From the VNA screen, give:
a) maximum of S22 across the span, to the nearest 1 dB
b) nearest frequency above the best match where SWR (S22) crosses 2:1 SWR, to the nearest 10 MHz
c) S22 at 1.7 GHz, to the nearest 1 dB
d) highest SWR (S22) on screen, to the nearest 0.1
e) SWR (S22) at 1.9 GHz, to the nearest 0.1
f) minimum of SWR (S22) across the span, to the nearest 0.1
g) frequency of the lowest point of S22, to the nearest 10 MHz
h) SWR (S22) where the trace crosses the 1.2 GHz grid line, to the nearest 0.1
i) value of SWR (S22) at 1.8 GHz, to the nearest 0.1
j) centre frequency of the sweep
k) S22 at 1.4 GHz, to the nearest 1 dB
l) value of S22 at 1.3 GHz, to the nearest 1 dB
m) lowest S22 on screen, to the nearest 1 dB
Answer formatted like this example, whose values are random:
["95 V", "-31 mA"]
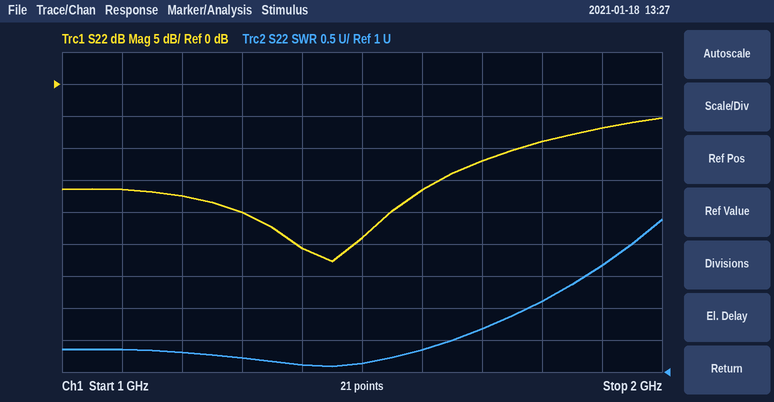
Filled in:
["-5 dB", "1.78 GHz", "-12 dB", "3.4", "2.7", "1.1", "1.45 GHz", "1.3", "2.1", "1.5 GHz", "-26 dB", "-20 dB", "-28 dB"]
